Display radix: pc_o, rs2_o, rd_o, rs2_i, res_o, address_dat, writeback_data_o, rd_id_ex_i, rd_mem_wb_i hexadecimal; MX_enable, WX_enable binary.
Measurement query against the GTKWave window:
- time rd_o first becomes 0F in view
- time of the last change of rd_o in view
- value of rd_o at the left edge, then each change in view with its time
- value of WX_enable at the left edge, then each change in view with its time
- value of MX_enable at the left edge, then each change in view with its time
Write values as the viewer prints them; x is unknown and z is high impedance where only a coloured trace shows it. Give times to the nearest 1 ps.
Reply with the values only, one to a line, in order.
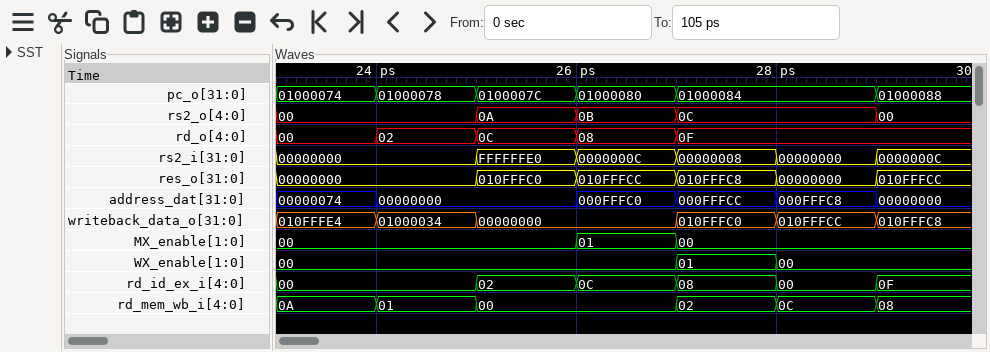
27 ps
27 ps
00, 02 at 24 ps, 0C at 25 ps, 08 at 26 ps, 0F at 27 ps
00, 01 at 27 ps, 00 at 28 ps
00, 01 at 26 ps, 00 at 27 ps
